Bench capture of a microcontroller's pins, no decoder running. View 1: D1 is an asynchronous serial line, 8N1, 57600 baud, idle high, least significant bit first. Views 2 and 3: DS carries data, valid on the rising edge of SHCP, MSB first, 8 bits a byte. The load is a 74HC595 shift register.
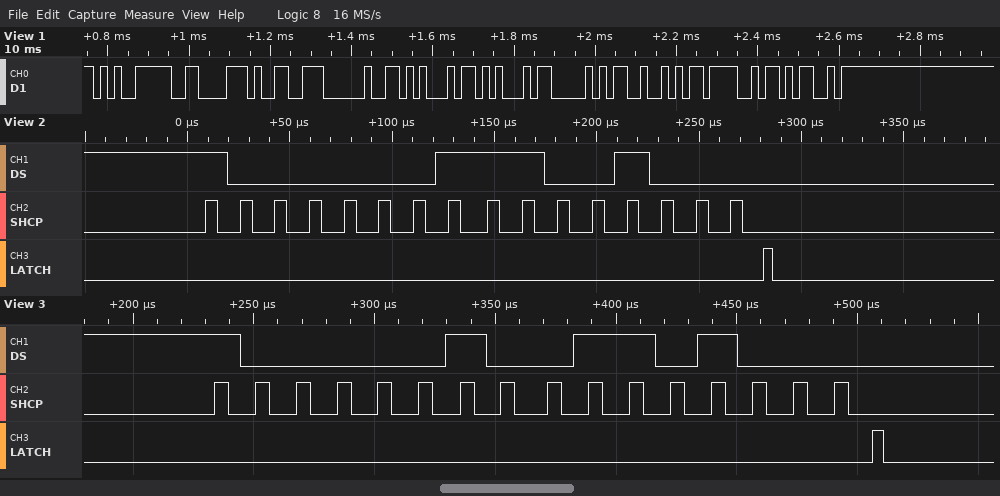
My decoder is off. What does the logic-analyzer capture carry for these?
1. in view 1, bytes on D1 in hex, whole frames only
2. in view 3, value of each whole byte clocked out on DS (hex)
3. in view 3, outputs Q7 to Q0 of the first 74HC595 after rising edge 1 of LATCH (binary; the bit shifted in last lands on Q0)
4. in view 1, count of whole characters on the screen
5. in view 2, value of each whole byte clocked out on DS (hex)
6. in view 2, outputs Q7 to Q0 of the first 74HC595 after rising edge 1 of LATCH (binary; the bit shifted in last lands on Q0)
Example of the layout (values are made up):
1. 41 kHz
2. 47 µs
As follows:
1. E5 86 99 20 45 45 50 52 4F 4D
2. 82 68
3. 01101000
4. 10
5. 81 C8
6. 11001000
